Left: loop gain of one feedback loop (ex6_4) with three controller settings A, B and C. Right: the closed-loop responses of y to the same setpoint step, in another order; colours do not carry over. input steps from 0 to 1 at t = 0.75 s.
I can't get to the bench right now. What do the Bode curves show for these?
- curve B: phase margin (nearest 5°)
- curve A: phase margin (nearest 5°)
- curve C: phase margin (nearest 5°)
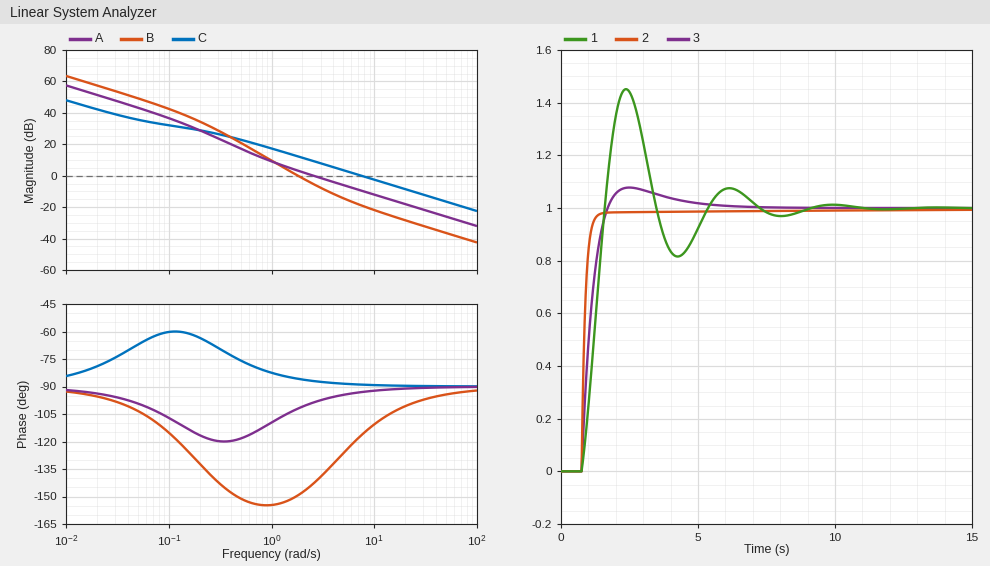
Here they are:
30°
80°
90°
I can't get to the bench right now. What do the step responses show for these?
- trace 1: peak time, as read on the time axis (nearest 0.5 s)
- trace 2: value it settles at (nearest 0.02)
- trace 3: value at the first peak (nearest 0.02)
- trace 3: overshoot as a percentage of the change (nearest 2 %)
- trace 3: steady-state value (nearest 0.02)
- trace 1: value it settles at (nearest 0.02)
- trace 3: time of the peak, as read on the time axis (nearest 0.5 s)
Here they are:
2.5 s
1.00
1.08
8 %
1.00
1.00
2.5 s
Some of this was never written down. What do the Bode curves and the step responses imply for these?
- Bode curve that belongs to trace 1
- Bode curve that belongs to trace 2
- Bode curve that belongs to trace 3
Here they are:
B
C
A
